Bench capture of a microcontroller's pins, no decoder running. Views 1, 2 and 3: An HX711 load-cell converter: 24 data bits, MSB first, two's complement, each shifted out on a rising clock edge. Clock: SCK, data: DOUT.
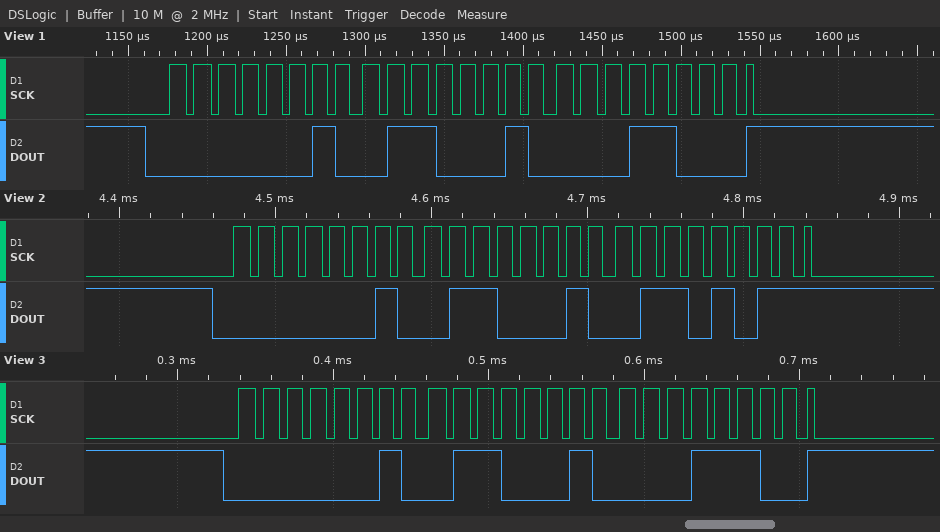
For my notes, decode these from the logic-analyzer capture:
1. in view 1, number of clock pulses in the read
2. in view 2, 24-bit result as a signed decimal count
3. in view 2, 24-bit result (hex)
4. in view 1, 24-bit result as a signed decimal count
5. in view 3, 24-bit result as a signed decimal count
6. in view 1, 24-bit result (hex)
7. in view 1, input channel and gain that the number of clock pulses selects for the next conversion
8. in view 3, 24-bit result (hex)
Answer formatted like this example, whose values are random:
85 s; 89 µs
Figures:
25; 156267; 0x02626B; 156184; 156188; 0x026218; channel A, gain 128; 0x02621C
